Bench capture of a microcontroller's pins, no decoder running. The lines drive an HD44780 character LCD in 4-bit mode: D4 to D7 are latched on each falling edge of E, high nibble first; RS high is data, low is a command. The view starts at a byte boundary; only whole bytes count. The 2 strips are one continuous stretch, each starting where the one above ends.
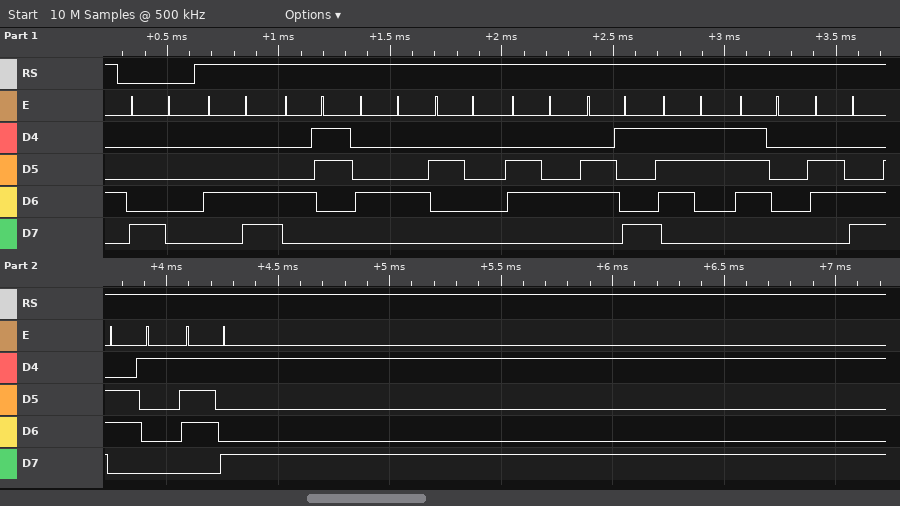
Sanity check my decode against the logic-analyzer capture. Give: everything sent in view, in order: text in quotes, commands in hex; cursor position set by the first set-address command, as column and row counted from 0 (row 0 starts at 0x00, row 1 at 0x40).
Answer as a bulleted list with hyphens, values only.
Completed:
- 0x80 "LCD display"
- column 0, row 0
